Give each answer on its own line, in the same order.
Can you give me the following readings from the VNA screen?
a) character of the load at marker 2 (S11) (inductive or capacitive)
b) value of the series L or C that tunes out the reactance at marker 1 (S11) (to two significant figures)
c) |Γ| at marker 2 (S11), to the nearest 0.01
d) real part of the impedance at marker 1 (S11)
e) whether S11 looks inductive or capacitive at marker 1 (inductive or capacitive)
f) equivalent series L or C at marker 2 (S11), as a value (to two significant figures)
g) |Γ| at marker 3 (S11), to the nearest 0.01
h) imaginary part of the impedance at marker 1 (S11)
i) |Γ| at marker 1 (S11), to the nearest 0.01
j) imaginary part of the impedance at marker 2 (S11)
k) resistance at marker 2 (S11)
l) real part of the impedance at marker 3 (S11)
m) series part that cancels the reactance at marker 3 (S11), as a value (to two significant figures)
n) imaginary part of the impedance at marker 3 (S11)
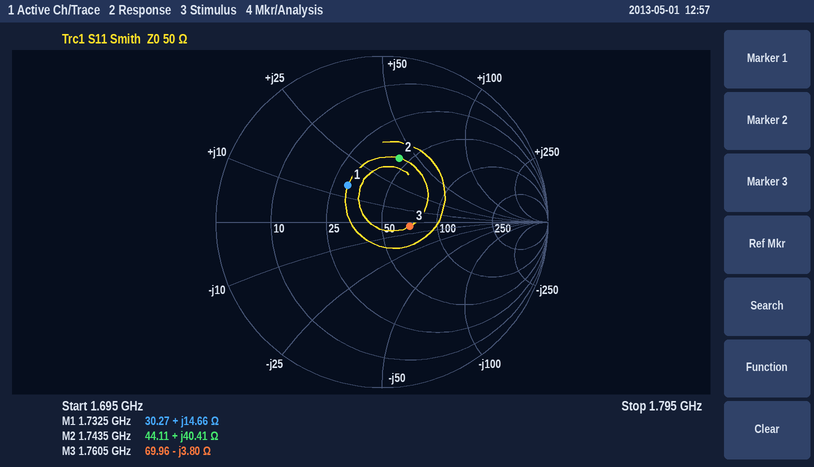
inductive
6.3 pF
0.40
30.27 Ω
inductive
3.7 nH
0.17
+14.66 Ω
0.30
+40.41 Ω
44.11 Ω
69.96 Ω
340 pH
-3.80 Ω
